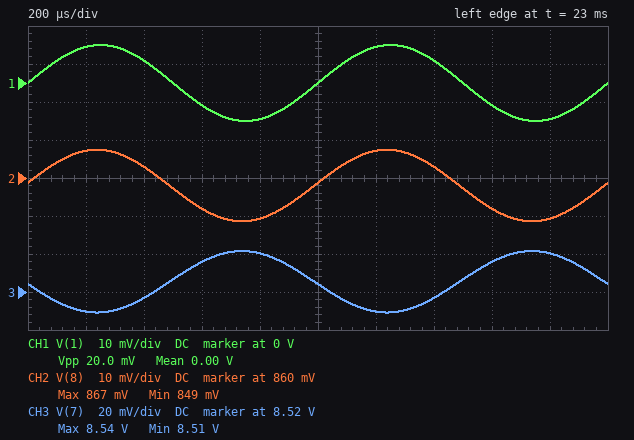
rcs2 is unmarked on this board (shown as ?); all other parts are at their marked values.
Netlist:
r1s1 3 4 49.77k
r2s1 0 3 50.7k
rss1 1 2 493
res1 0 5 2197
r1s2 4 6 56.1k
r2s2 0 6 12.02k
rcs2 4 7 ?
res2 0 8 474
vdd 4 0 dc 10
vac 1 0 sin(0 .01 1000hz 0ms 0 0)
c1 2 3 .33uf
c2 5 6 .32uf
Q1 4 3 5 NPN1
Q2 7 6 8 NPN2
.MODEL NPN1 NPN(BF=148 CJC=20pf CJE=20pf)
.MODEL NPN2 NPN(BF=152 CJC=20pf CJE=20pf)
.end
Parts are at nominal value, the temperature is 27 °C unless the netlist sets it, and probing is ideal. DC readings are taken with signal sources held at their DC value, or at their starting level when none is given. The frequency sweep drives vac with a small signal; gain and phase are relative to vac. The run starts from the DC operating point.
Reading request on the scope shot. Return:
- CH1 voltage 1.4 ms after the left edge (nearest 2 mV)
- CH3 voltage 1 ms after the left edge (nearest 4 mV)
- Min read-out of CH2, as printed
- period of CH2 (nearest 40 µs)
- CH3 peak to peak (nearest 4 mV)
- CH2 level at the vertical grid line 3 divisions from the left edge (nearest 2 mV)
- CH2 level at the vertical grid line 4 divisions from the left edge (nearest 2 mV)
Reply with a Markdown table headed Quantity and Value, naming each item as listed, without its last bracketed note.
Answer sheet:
| Quantity | Value |
|---|---|
| CH1 voltage 1.4 ms after the left edge | 6 mV |
| CH3 voltage 1 ms after the left edge | 8.524 V |
| Min read-out of CH2, as printed | 849 mV |
| period of CH2 | 1.00 ms |
| CH3 peak to peak | 32 mV |
| CH2 level at the vertical grid line 3 divisions from the left edge | 852 mV |
| CH2 level at the vertical grid line 4 divisions from the left edge | 850 mV |
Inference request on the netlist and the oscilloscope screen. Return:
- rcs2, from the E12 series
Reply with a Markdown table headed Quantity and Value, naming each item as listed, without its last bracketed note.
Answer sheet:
| Quantity | Value |
|---|---|
| rcs2, from the E12 series | 820 Ω |
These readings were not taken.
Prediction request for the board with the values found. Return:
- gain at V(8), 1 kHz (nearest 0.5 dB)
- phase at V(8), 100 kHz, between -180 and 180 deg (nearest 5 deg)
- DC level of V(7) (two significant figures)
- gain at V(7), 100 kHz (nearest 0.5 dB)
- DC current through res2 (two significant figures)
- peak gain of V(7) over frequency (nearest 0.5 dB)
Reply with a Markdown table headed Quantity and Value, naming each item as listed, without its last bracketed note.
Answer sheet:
| Quantity | Value |
|---|---|
| gain at V(8), 1 kHz | -0.5 dB |
| phase at V(8), 100 kHz, between -180 and 180 deg | 0 deg |
| DC level of V(7) | 8.5 V |
| gain at V(7), 100 kHz | 4.0 dB |
| DC current through res2 | 1.8 mA |
| peak gain of V(7) over frequency | 4.0 dB |
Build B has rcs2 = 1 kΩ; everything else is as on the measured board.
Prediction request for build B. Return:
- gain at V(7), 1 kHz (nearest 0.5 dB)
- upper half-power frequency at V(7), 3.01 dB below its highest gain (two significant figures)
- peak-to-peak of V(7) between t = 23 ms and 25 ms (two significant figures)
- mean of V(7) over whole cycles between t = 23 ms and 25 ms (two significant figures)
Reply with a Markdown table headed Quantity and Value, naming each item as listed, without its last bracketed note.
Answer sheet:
| Quantity | Value |
|---|---|
| gain at V(7), 1 kHz | 6.0 dB |
| upper half-power frequency at V(7), 3.01 dB below its highest gain | 16 MHz |
| peak-to-peak of V(7) between t = 23 ms and 25 ms | 39 mV |
| mean of V(7) over whole cycles between t = 23 ms and 25 ms | 8.2 V |
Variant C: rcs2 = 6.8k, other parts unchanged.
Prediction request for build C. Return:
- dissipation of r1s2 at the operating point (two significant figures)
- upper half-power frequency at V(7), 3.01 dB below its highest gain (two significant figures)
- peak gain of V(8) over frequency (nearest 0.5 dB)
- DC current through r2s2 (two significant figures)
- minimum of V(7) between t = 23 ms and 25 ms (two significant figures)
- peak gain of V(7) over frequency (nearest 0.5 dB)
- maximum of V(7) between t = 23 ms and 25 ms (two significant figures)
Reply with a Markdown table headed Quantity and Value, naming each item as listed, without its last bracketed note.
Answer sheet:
| Quantity | Value |
|---|---|
| dissipation of r1s2 at the operating point | 1.3 mW |
| upper half-power frequency at V(7), 3.01 dB below its highest gain | 31 MHz |
| peak gain of V(8) over frequency | -1.0 dB |
| DC current through r2s2 | 120 µA |
| minimum of V(7) between t = 23 ms and 25 ms | 760 mV |
| peak gain of V(7) over frequency | -0.5 dB |
| maximum of V(7) between t = 23 ms and 25 ms | 780 mV |
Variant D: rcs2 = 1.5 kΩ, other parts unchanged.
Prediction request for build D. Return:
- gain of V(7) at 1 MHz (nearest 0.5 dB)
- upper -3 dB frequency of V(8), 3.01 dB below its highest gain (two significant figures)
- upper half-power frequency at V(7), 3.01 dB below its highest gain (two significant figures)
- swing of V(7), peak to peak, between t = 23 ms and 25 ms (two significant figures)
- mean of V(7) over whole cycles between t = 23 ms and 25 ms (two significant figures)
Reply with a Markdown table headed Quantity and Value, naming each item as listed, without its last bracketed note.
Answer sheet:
| Quantity | Value |
|---|---|
| gain of V(7) at 1 MHz | 9.5 dB |
| upper -3 dB frequency of V(8), 3.01 dB below its highest gain | 27 MHz |
| upper half-power frequency at V(7), 3.01 dB below its highest gain | 11 MHz |
| swing of V(7), peak to peak, between t = 23 ms and 25 ms | 59 mV |
| mean of V(7) over whole cycles between t = 23 ms and 25 ms | 7.3 V |
